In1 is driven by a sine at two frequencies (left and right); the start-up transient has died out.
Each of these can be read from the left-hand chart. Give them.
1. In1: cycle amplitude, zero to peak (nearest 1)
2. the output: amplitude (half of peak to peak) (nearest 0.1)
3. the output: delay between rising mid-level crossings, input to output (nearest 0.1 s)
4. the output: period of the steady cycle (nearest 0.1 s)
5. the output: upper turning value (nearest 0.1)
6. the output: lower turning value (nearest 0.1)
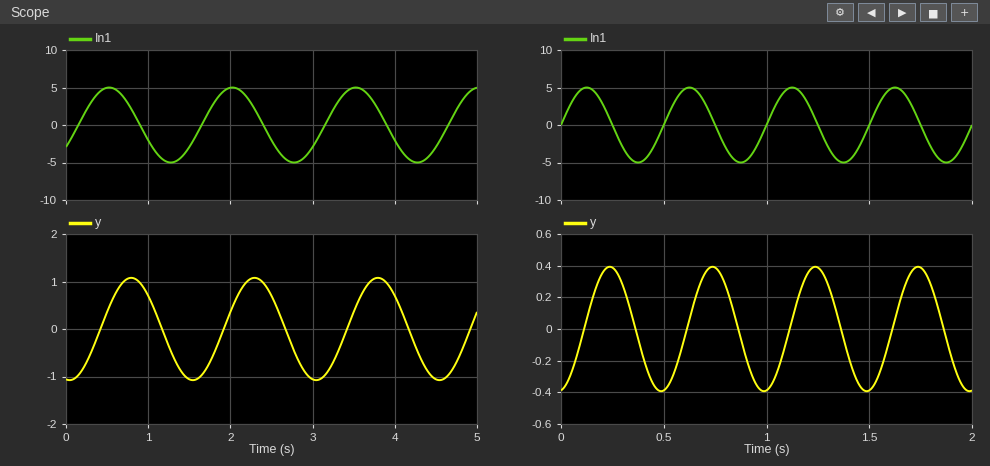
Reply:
5
1.1
0.3 s
1.5 s
1.1
-1.1
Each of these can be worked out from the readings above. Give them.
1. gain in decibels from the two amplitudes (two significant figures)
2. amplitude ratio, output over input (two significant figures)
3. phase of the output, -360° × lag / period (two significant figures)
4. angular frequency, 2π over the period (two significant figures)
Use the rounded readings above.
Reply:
-13 dB
0.22
-72°
4.2 rad/s
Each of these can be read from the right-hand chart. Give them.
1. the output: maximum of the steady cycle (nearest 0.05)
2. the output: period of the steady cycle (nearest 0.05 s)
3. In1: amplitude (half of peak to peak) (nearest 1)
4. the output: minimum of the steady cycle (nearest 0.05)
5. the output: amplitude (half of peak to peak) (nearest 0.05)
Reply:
0.40
0.50 s
5
-0.40
0.40
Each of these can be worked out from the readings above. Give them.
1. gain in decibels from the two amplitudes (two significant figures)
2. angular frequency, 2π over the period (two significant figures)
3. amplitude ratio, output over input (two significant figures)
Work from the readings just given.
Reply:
-22 dB
13 rad/s
0.080
